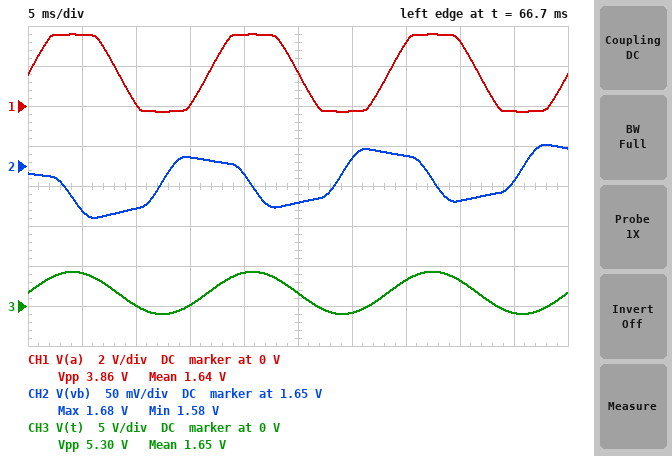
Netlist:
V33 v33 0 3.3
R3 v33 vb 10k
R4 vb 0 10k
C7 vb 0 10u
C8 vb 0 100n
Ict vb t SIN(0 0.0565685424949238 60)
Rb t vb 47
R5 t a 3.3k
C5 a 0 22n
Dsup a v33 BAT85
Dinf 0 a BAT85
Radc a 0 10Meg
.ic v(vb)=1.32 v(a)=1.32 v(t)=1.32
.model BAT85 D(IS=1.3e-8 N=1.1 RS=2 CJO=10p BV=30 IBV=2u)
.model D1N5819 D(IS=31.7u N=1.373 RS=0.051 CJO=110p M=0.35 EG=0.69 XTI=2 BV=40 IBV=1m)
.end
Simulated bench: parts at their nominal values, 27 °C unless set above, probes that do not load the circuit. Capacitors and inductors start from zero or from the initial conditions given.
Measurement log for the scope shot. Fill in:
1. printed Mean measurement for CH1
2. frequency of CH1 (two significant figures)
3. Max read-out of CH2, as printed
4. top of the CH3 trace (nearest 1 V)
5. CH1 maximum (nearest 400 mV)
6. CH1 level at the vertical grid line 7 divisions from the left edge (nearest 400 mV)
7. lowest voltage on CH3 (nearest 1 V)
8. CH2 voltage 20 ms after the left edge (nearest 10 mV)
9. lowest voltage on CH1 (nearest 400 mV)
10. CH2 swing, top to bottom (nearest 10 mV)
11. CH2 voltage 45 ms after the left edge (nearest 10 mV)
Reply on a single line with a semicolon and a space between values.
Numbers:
1.64 V; 60 Hz; 1.68 V; 4 V; 3.6 V; 3.2 V; -1 V; 1.64 V; -400 mV; 90 mV; 1.63 V
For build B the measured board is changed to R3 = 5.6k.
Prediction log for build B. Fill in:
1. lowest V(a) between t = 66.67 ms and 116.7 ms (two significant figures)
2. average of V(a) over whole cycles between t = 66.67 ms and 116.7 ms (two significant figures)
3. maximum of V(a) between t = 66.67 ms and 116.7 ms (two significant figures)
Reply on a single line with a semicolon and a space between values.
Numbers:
-260 mV; 1.8 V; 3.6 V
